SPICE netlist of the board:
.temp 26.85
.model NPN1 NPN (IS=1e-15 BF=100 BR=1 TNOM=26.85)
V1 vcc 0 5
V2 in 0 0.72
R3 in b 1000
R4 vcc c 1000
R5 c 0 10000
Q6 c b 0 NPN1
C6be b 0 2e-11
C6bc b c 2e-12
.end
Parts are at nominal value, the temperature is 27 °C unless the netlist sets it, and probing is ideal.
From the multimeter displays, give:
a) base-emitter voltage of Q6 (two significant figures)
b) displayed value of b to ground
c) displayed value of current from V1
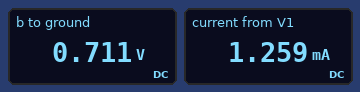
710 mV
0.711 V
1.259 mA
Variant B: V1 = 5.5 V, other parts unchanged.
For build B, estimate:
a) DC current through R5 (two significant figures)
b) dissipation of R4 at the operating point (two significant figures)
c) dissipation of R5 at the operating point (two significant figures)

420 µA
1.7 mW
1.8 mW
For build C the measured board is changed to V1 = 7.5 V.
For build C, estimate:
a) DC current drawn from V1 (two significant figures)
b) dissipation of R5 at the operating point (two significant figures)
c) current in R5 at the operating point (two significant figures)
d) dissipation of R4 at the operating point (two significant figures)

1.5 mA
3.6 mW
600 µA
2.2 mW
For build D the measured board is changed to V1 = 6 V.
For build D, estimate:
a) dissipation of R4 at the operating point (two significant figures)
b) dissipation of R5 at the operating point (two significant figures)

1.8 mW
2.2 mW
